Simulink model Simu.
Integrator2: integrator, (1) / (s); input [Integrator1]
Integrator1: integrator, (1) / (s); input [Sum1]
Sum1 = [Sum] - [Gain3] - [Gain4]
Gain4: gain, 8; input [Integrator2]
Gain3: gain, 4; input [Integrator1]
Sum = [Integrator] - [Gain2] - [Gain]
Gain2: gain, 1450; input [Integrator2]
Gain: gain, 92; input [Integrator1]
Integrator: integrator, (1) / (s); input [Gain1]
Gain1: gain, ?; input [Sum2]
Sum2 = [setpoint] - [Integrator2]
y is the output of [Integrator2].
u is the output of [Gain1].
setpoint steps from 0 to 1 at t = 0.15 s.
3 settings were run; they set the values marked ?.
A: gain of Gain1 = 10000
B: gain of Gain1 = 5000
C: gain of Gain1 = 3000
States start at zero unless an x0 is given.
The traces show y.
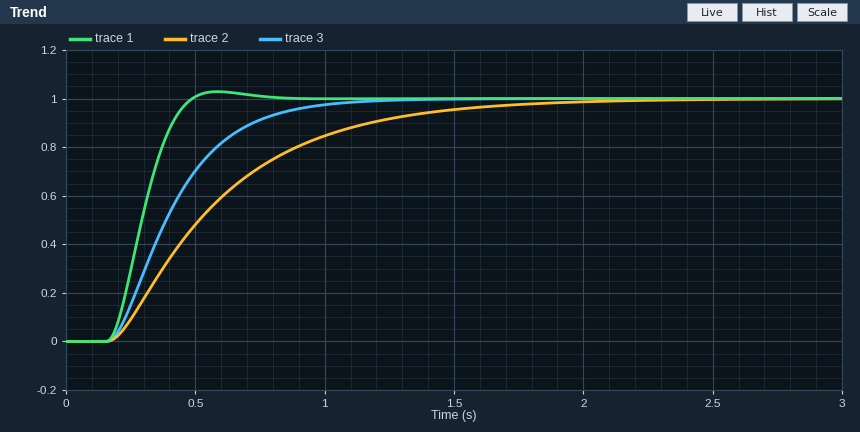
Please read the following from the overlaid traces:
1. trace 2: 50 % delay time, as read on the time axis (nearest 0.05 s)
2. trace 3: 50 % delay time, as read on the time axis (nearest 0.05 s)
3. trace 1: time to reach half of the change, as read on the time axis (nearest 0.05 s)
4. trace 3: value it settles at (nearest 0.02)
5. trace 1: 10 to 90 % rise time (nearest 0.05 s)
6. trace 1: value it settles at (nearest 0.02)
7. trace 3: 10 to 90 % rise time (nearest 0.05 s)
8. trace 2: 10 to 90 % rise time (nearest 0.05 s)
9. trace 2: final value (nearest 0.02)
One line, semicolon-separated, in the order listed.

0.50 s; 0.40 s; 0.30 s; 1.00; 0.20 s; 1.00; 0.50 s; 0.90 s; 1.00
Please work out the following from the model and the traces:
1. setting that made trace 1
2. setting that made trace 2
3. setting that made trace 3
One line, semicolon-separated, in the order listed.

A; C; B
